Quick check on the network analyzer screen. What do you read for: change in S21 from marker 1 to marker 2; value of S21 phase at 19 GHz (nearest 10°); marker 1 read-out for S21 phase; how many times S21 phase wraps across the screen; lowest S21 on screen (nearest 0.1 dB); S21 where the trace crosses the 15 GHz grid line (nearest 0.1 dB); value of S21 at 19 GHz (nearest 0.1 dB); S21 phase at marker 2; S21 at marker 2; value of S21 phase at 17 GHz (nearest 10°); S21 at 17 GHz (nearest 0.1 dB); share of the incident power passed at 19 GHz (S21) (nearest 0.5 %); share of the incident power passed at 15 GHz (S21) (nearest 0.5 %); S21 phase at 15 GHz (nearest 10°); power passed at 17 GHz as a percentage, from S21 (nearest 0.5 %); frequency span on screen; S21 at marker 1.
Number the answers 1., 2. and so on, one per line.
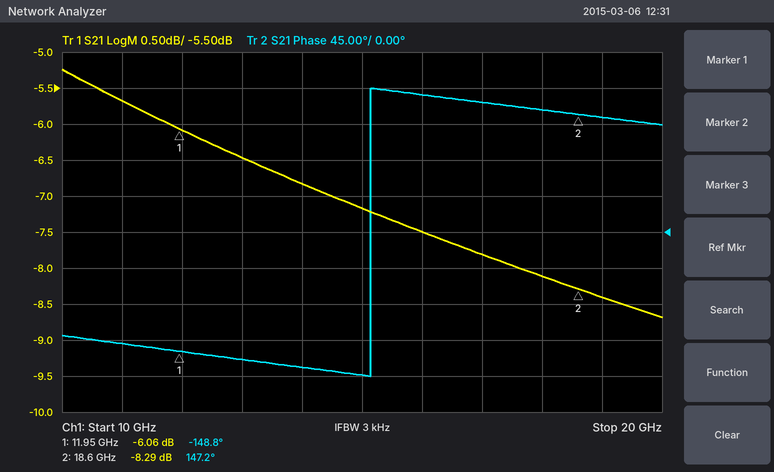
1. -2.23 dB
2. 140°
3. -148.8°
4. 1
5. -8.7 dB
6. -7.2 dB
7. -8.4 dB
8. 147.2°
9. -8.29 dB
10. 160°
11. -7.8 dB
12. 14.5 %
13. 19.0 %
14. -180°
15. 16.5 %
16. 10 GHz
17. -6.06 dB
